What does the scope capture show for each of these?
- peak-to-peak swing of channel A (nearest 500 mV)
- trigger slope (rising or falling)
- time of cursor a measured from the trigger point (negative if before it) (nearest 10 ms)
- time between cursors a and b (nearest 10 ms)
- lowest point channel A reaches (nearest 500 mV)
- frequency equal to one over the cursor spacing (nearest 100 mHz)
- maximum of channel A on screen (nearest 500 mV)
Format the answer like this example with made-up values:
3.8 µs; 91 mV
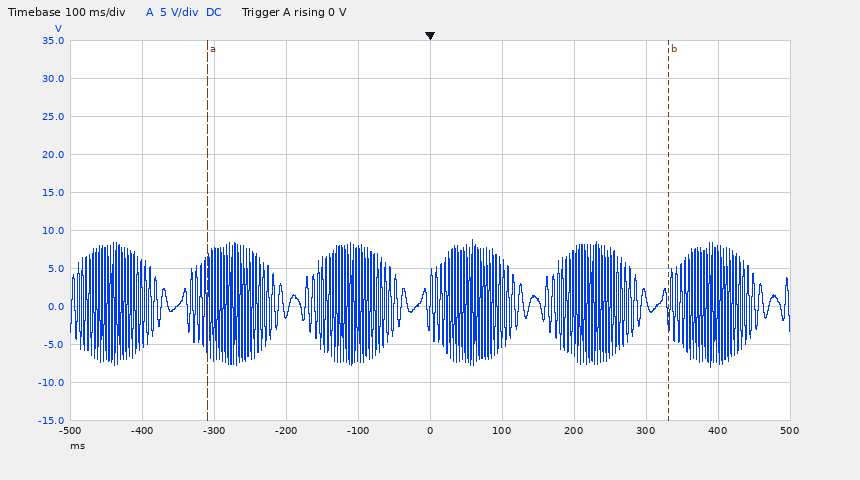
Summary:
17.0 V; rising; -310 ms; 640 ms; -8.0 V; 1.6 Hz; 9.0 V
